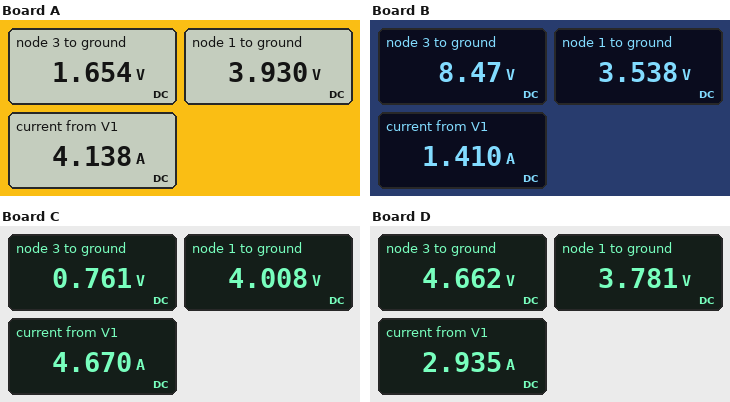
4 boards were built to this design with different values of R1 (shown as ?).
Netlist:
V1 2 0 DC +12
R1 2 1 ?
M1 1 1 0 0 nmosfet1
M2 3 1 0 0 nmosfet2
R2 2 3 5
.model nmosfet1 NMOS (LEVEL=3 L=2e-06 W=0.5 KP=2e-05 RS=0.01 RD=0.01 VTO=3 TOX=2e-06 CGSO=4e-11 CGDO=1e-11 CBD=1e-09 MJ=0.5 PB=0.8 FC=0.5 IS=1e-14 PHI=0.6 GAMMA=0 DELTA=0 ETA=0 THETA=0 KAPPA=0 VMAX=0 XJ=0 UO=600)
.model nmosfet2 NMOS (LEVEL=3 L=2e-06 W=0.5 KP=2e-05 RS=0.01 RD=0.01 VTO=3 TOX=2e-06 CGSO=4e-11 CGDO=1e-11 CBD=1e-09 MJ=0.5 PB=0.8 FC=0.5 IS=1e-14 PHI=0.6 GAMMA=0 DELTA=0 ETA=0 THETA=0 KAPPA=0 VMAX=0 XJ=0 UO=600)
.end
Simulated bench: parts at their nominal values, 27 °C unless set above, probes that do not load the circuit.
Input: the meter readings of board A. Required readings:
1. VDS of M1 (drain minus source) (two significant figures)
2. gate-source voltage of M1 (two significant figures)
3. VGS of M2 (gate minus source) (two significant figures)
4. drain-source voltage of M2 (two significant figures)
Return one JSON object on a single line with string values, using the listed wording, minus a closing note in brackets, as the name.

{"VDS of M1 (drain minus source)": "3.9 V", "gate-source voltage of M1": "3.9 V", "VGS of M2 (gate minus source)": "3.9 V", "drain-source voltage of M2": "1.7 V"}
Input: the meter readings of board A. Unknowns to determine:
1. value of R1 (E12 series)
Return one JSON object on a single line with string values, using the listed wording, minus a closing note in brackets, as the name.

{"value of R1": "3.9 Ω"}
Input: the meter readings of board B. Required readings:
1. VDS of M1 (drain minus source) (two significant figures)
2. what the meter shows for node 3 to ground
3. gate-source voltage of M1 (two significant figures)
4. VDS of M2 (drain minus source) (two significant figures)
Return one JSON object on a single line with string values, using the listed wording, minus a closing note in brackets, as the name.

{"VDS of M1 (drain minus source)": "3.5 V", "what the meter shows for node 3 to ground": "8.47 V", "gate-source voltage of M1": "3.5 V", "VDS of M2 (drain minus source)": "8.5 V"}
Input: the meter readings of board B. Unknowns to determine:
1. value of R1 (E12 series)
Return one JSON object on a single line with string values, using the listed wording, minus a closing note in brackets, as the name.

{"value of R1": "12 Ω"}
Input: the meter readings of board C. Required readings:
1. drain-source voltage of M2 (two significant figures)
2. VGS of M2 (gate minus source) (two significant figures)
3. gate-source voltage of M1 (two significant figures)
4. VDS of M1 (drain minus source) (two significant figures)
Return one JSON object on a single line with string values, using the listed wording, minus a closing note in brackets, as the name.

{"drain-source voltage of M2": "760 mV", "VGS of M2 (gate minus source)": "4.0 V", "gate-source voltage of M1": "4.0 V", "VDS of M1 (drain minus source)": "4.0 V"}
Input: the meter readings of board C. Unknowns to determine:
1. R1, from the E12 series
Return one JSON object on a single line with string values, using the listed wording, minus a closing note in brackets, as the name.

{"R1, from the E12 series": "3.3 Ω"}
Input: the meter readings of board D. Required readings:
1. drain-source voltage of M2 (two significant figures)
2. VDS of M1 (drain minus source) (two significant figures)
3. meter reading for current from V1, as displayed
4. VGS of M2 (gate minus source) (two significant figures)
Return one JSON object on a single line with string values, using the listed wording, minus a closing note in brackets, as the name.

{"drain-source voltage of M2": "4.7 V", "VDS of M1 (drain minus source)": "3.8 V", "meter reading for current from V1, as displayed": "2.935 A", "VGS of M2 (gate minus source)": "3.8 V"}
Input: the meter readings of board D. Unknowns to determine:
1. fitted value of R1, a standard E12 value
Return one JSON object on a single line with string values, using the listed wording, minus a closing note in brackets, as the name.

{"fitted value of R1, a standard E12 value": "5.6 Ω"}
